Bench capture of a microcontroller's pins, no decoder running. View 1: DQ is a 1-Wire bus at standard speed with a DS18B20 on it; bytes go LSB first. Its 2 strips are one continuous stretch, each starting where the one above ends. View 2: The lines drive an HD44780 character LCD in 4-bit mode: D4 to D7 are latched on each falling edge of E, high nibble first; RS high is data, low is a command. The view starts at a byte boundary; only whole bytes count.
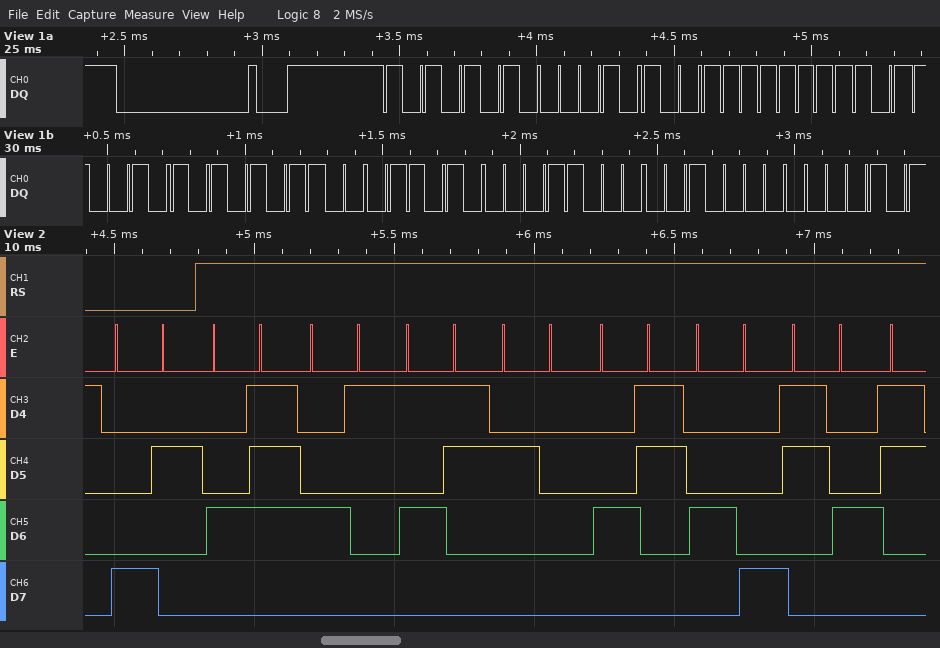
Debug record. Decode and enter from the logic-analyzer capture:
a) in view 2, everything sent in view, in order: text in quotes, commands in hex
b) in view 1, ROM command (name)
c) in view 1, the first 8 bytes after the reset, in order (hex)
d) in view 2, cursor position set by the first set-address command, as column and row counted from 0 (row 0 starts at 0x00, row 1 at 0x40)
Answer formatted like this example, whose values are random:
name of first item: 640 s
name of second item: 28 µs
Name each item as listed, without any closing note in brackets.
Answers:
in view 2, everything sent in view, in order: text in quotes, commands in hex: 0x82 "GAS CH4"
in view 1, ROM command: Match ROM
in view 1, the first 8 bytes after the reset, in order: 55 28 FF 4D D5 58 18 04
in view 2, cursor position set by the first set-address command, as column and row counted from 0: column 2, row 0
